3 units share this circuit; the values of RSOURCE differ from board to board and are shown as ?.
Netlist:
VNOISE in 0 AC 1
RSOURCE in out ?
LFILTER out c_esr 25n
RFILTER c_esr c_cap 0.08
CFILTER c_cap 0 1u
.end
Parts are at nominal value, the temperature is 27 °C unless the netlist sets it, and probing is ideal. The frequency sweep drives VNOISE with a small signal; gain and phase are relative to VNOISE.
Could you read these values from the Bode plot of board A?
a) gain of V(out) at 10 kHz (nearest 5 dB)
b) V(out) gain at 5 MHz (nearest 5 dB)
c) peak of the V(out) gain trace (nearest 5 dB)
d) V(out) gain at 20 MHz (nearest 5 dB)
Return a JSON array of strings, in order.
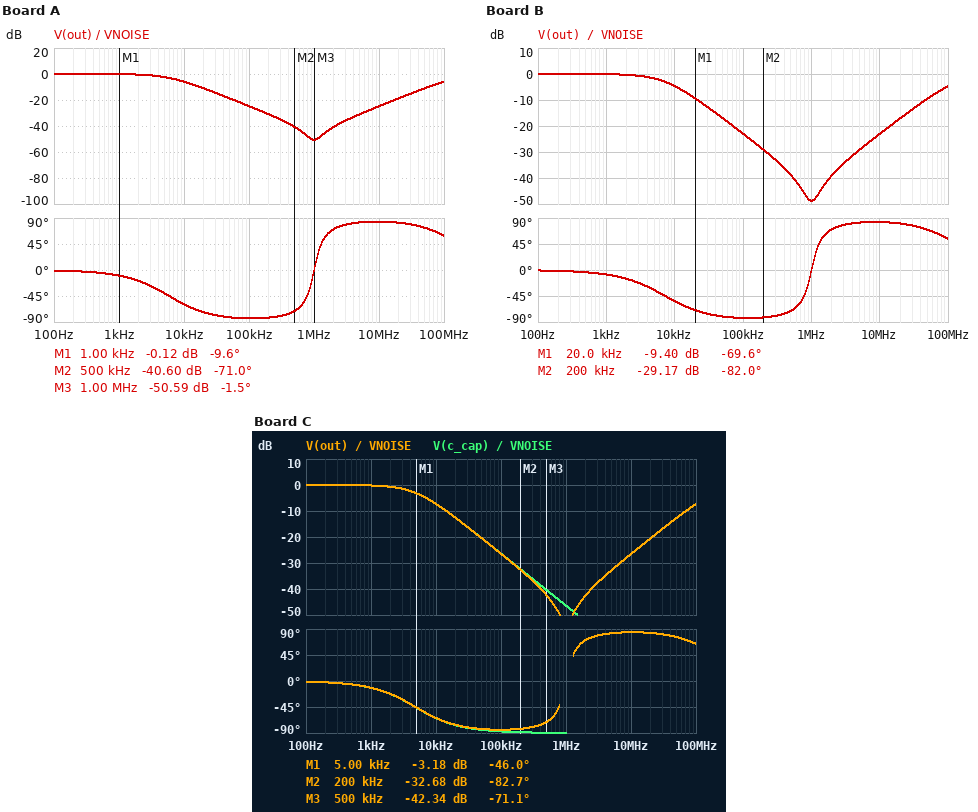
["-5 dB", "-30 dB", "0 dB", "-20 dB"]
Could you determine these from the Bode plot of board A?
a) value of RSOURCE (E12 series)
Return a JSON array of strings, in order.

["27 Ω"]
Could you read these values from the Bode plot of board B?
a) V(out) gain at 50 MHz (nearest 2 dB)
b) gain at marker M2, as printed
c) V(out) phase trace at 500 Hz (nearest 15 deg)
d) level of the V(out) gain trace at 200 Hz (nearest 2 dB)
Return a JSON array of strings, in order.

["-10 dB", "-29.17 dB", "0 deg", "0 dB"]
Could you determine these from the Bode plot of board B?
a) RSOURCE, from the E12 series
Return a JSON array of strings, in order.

["22 Ω"]
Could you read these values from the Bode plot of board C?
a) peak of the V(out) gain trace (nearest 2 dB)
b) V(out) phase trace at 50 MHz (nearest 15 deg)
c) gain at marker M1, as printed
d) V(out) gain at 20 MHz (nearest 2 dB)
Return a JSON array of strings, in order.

["0 dB", "75 deg", "-3.18 dB", "-20 dB"]
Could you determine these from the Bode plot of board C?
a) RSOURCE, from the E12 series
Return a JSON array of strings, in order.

["33 Ω"]
